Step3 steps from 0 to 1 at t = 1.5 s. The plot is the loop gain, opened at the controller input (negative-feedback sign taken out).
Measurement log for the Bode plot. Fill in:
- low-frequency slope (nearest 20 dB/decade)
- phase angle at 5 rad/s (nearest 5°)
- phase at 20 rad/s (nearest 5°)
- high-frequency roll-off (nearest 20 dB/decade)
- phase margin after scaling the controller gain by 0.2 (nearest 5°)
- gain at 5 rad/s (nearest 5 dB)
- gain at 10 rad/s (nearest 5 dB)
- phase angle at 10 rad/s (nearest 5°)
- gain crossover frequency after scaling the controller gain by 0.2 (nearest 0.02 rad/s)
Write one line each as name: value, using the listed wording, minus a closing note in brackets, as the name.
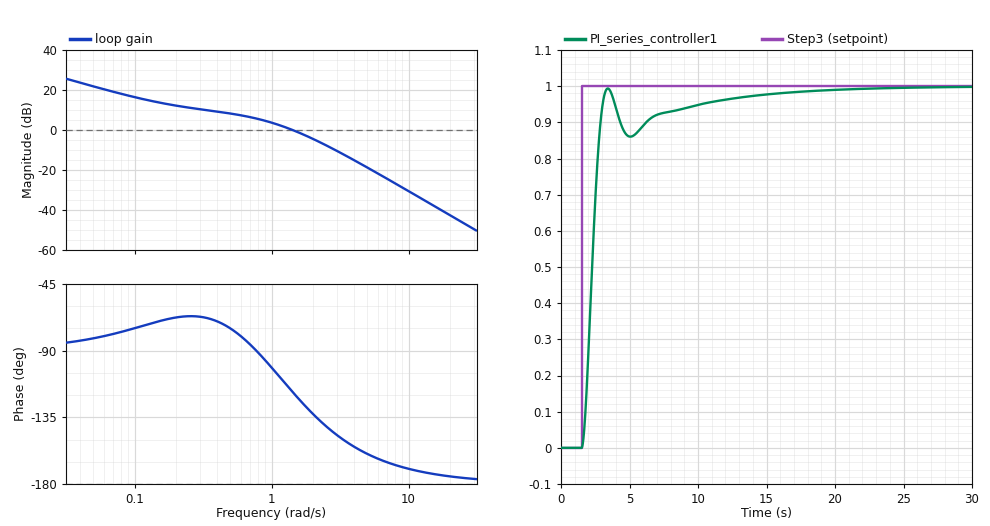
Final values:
low-frequency slope: -20 dB/decade
phase angle at 5 rad/s: -160°
phase at 20 rad/s: -175°
high-frequency roll-off: -40 dB/decade
phase margin after scaling the controller gain by 0.2: 110°
gain at 5 rad/s: -20 dB
gain at 10 rad/s: -30 dB
phase angle at 10 rad/s: -170°
gain crossover frequency after scaling the controller gain by 0.2: 0.14 rad/s
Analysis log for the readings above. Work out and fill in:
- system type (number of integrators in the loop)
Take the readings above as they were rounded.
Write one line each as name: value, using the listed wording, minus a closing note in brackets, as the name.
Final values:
system type: 1
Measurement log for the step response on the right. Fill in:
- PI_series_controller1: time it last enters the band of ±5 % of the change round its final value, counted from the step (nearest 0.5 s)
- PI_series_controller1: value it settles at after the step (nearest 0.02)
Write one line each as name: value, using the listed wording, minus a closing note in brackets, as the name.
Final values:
PI_series_controller1: time it last enters the band of ±5 % of the change round its final value, counted from the step: 8.5 s
PI_series_controller1: value it settles at after the step: 1.00
